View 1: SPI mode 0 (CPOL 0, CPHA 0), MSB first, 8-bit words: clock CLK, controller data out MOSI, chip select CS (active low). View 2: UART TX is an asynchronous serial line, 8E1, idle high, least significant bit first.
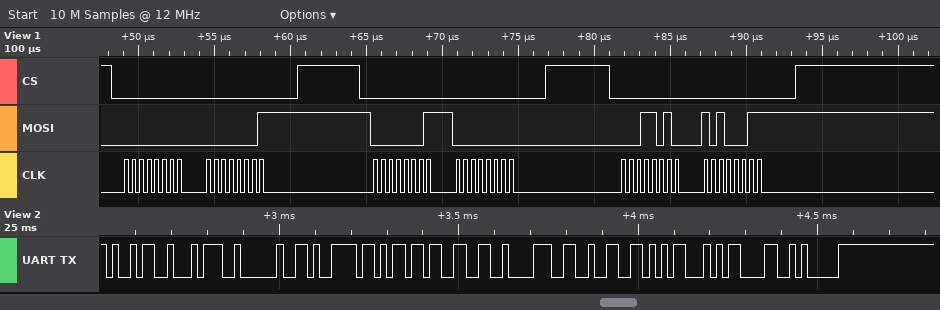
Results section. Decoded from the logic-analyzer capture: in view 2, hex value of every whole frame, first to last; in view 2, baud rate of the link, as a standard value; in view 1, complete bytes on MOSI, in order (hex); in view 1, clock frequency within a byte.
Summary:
69 74 20 79 6D 66 38 32 35 0D 0A
57600 baud
0x00 0x01 0x01 0x00 0x1A 0xA3
2 MHz
